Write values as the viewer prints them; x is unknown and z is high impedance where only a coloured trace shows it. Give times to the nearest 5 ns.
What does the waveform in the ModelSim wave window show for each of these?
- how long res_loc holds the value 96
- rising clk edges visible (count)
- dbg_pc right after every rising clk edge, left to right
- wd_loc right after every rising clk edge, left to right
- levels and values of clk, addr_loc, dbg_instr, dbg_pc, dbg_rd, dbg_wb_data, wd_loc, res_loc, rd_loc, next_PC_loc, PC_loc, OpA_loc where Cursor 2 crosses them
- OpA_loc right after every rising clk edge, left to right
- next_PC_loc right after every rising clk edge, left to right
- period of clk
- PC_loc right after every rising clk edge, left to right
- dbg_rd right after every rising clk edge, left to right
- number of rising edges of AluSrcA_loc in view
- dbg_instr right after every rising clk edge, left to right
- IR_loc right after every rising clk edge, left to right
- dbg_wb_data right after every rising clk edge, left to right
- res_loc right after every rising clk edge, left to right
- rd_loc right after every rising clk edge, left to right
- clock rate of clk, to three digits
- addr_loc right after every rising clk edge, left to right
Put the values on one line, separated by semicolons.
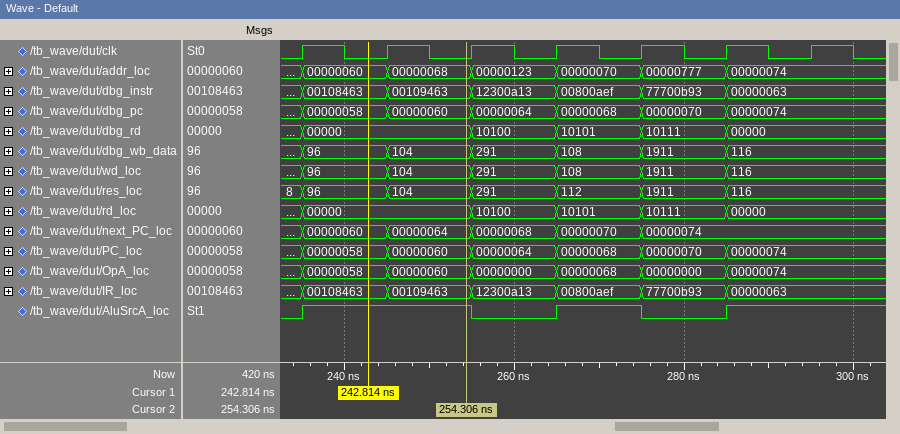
10 ns; 7; 00000058, 00000060, 00000064, 00000068, 00000070, 00000074, 00000074; 96, 104, 291, 108, 1911, 116, 116; clk=0, addr_loc=00000068, dbg_instr=00109463, dbg_pc=00000060, dbg_rd=00000, dbg_wb_data=104, wd_loc=104, res_loc=104, rd_loc=00000, next_PC_loc=00000064, PC_loc=00000060, OpA_loc=00000060; 00000058, 00000060, 00000000, 00000068, 00000000, 00000074, 00000074; 00000060, 00000064, 00000068, 00000070, 00000074, 00000074, 00000074; 10 ns; 00000058, 00000060, 00000064, 00000068, 00000070, 00000074, 00000074; 00000, 00000, 10100, 10101, 10111, 00000, 00000; 3; 00108463, 00109463, 12300a13, 00800aef, 77700b93, 00000063, 00000063; 00108463, 00109463, 12300a13, 00800aef, 77700b93, 00000063, 00000063; 96, 104, 291, 108, 1911, 116, 116; 96, 104, 291, 112, 1911, 116, 116; 00000, 00000, 10100, 10101, 10111, 00000, 00000; 100 MHz; 00000060, 00000068, 00000123, 00000070, 00000777, 00000074, 00000074
